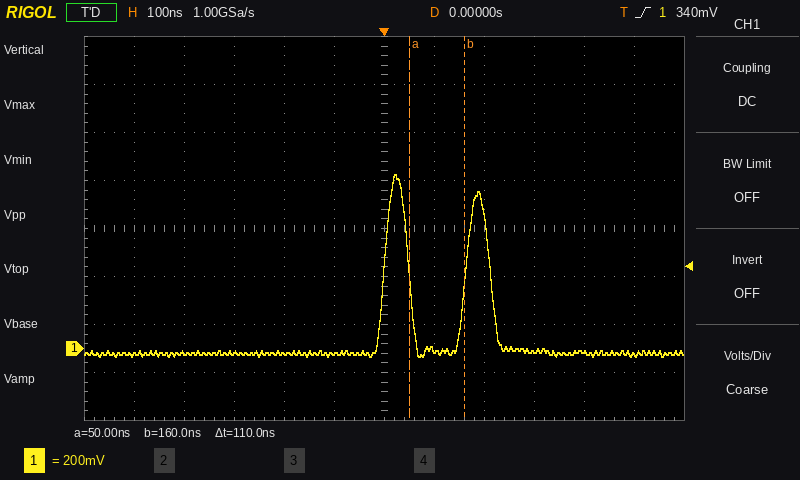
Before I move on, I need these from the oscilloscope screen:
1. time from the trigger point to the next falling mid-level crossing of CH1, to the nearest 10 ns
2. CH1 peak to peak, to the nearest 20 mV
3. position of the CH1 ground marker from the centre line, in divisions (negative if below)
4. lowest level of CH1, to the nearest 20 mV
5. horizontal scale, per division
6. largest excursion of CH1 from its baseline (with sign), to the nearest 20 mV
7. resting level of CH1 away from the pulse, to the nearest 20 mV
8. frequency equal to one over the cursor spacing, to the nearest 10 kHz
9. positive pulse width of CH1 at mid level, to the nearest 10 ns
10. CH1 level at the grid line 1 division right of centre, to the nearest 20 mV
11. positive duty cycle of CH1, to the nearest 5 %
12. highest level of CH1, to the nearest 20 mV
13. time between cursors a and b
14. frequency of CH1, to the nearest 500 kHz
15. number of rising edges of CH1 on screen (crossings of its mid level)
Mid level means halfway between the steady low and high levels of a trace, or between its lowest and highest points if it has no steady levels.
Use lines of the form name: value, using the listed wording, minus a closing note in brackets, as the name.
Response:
time from the trigger point to the next falling mid-level crossing of CH1, to the nearest 10 ns: 50 ns
CH1 peak to peak, to the nearest 20 mV: 760 mV
position of the CH1 ground marker from the centre line, in divisions: -2.5 div
lowest level of CH1, to the nearest 20 mV: -40 mV
horizontal scale, per division: 100 ns
largest excursion of CH1 from its baseline (with sign), to the nearest 20 mV: +740 mV
resting level of CH1 away from the pulse, to the nearest 20 mV: -20 mV
frequency equal to one over the cursor spacing, to the nearest 10 kHz: 9.09 MHz
positive pulse width of CH1 at mid level, to the nearest 10 ns: 50 ns
CH1 level at the grid line 1 division right of centre, to the nearest 20 mV: 0 mV
positive duty cycle of CH1, to the nearest 5 %: 30 %
highest level of CH1, to the nearest 20 mV: 720 mV
time between cursors a and b: 110 ns
frequency of CH1, to the nearest 500 kHz: 6.0 MHz
number of rising edges of CH1 on screen: 2
